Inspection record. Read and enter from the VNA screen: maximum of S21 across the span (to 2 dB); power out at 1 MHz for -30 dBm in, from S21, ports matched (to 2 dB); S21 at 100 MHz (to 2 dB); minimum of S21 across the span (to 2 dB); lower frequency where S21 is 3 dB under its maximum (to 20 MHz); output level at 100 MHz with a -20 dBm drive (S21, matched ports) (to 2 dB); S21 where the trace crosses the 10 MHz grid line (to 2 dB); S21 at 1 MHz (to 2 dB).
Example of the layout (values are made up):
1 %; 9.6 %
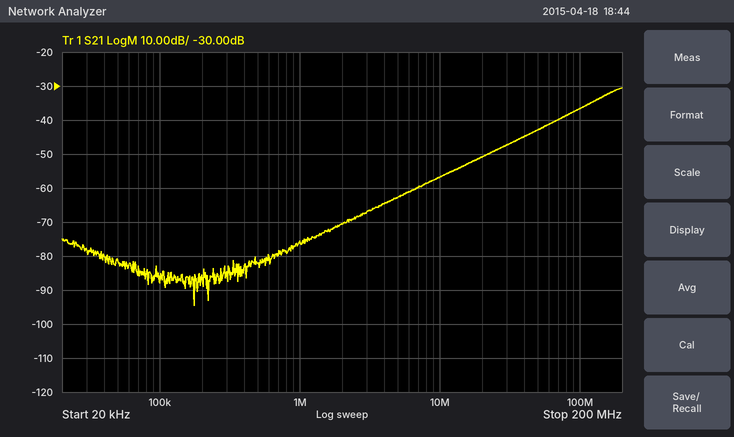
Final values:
-30 dB; -106 dBm; -36 dB; -94 dB; 140 MHz; -56 dBm; -56 dB; -76 dB
